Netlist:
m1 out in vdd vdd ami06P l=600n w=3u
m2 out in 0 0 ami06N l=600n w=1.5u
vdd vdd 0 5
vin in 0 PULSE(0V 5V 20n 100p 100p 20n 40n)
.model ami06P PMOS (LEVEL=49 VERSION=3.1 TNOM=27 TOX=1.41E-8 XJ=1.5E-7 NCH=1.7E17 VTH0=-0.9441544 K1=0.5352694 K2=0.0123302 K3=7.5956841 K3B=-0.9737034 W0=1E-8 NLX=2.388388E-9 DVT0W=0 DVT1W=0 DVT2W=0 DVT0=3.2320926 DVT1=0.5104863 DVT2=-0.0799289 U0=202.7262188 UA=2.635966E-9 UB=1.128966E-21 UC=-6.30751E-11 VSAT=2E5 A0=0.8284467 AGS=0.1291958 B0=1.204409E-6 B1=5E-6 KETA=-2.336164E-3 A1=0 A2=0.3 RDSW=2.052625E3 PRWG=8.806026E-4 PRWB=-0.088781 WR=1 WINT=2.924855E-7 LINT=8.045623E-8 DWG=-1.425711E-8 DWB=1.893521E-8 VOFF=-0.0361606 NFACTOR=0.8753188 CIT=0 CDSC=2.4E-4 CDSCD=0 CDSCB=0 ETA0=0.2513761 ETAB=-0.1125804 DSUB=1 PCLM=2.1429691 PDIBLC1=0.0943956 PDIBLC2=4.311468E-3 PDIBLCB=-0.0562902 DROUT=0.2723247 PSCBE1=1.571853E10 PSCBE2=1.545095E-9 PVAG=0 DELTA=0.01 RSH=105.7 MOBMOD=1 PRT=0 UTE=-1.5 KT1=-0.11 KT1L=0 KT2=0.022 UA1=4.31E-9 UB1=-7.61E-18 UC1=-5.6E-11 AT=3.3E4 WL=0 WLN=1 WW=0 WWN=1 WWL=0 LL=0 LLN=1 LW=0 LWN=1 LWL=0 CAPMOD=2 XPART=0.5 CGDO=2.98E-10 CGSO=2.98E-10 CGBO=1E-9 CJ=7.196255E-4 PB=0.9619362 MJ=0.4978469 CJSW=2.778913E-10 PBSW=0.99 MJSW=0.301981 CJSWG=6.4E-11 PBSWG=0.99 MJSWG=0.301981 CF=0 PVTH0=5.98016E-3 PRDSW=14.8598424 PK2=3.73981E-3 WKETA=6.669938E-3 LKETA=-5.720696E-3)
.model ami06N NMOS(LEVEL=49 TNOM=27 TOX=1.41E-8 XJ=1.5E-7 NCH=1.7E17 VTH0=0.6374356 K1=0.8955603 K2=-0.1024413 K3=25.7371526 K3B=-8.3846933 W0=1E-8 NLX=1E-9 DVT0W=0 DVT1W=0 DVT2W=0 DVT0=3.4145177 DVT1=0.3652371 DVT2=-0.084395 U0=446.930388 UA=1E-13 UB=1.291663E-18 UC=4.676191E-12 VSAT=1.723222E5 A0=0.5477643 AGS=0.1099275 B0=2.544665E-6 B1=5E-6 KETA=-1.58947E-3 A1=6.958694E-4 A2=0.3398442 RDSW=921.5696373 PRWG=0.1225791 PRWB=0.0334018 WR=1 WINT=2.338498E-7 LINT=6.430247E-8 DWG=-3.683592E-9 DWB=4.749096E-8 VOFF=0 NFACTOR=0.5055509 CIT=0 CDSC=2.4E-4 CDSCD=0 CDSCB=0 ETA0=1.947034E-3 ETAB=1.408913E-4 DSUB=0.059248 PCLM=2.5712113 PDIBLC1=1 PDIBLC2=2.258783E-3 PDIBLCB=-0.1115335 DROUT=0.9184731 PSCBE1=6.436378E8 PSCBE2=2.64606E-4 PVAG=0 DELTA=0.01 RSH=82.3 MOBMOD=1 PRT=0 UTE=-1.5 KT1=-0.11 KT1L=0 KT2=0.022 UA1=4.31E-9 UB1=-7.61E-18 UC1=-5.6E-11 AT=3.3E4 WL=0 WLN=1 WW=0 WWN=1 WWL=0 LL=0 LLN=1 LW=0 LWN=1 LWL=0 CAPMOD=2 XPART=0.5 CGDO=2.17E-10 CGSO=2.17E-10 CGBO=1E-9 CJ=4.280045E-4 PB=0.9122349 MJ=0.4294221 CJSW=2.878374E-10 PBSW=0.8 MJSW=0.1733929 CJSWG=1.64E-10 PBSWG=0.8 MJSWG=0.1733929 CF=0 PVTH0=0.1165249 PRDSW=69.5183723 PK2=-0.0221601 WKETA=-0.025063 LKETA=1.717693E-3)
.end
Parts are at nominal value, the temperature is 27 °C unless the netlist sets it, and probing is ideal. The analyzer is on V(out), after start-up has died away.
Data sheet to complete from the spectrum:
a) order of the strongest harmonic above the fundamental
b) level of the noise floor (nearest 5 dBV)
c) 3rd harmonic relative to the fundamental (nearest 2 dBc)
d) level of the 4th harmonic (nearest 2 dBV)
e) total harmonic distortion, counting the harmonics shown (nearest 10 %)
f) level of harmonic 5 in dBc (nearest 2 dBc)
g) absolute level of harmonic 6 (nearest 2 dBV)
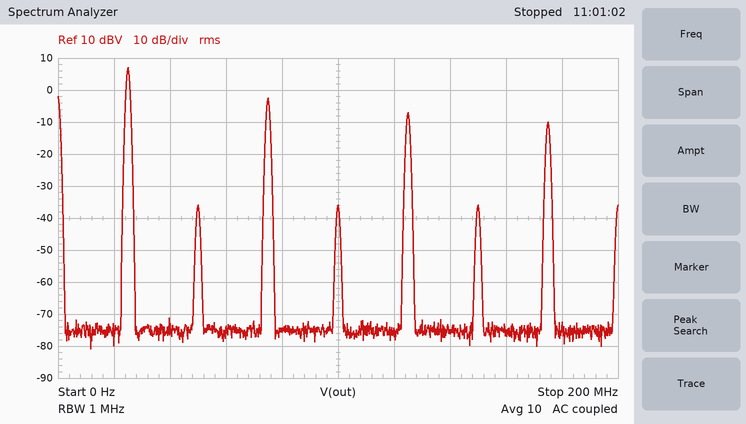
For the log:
3
-75 dBV
-10 dBc
-36 dBV
40 %
-14 dBc
-36 dBV
